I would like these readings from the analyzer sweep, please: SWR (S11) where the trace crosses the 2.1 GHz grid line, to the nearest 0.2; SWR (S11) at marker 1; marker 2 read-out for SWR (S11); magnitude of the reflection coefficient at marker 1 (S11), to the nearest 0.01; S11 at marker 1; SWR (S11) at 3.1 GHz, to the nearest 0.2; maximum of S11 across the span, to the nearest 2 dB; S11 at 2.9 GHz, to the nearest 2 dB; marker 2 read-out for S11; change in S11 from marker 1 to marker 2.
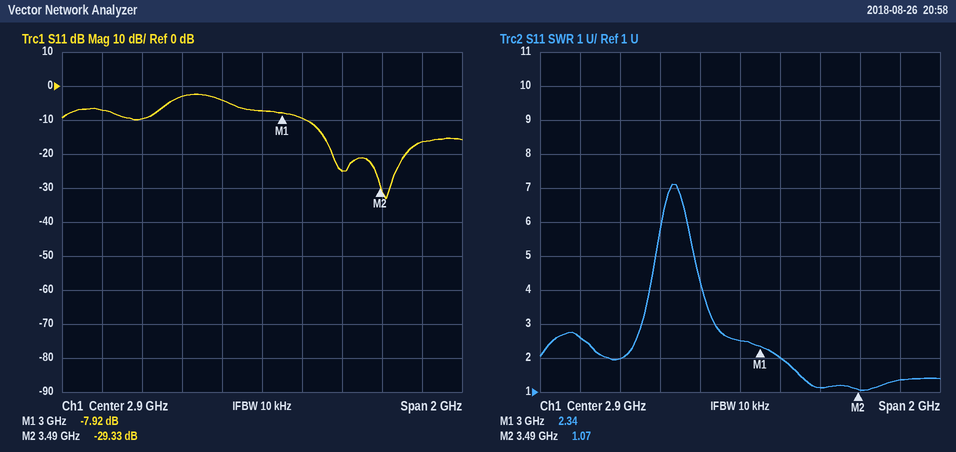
2.6
2.34
1.07
0.40
-7.92 dB
2.0
-2 dB
-8 dB
-29.33 dB
-21.41 dB
